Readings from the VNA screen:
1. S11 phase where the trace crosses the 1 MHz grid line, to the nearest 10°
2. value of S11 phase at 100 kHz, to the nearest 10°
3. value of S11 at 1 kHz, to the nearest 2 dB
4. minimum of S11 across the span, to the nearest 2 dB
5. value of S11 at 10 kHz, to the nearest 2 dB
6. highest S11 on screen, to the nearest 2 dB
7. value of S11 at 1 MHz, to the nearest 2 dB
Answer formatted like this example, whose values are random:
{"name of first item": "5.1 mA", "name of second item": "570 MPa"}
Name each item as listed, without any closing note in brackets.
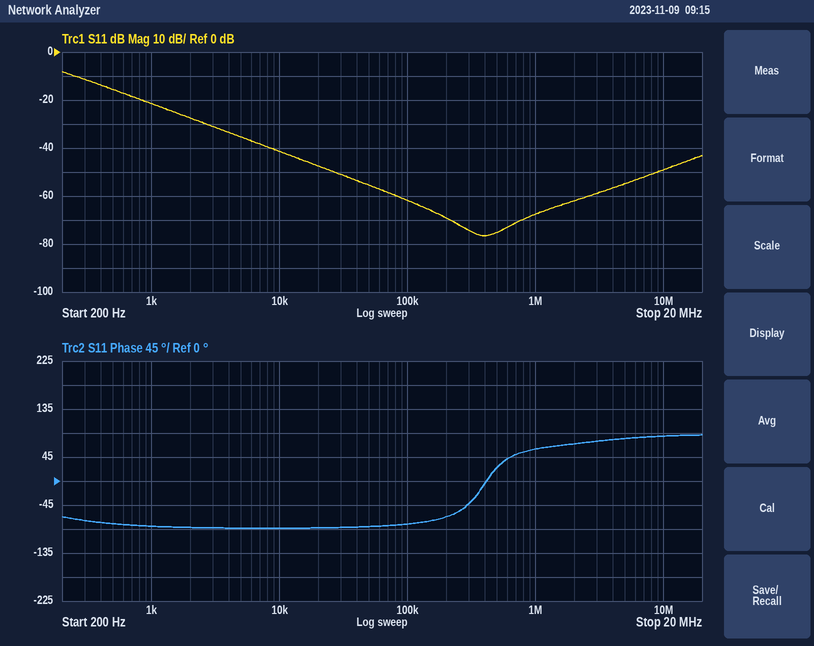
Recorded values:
{"S11 phase where the trace crosses the 1 MHz grid line, to the nearest 10°": "60°", "value of S11 phase at 100 kHz, to the nearest 10°": "-80°", "value of S11 at 1 kHz, to the nearest 2 dB": "-22 dB", "minimum of S11 across the span, to the nearest 2 dB": "-76 dB", "value of S11 at 10 kHz, to the nearest 2 dB": "-42 dB", "highest S11 on screen, to the nearest 2 dB": "-8 dB", "value of S11 at 1 MHz, to the nearest 2 dB": "-68 dB"}
